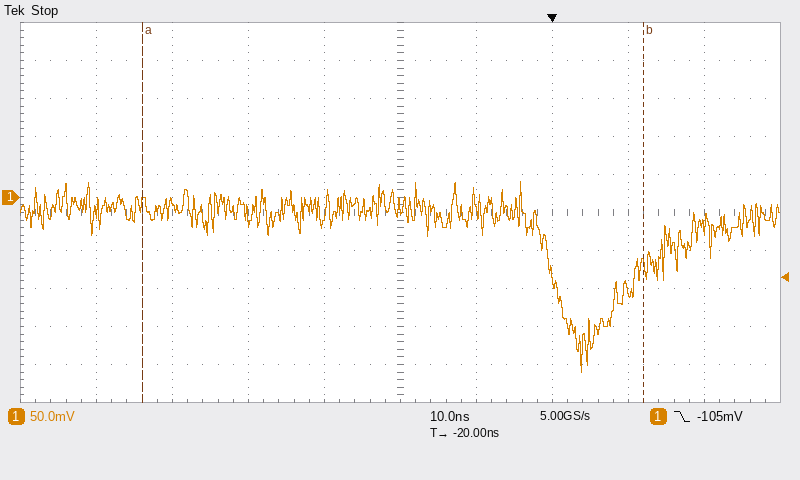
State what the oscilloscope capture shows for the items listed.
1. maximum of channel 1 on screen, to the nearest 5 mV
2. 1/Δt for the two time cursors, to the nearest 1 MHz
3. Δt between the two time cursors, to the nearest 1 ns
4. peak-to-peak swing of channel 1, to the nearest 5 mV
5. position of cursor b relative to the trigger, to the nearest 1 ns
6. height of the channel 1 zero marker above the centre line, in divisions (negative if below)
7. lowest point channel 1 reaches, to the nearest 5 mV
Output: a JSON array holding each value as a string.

["20 mV", "15 MHz", "66 ns", "250 mV", "+12 ns", "+0.4 div", "-230 mV"]
